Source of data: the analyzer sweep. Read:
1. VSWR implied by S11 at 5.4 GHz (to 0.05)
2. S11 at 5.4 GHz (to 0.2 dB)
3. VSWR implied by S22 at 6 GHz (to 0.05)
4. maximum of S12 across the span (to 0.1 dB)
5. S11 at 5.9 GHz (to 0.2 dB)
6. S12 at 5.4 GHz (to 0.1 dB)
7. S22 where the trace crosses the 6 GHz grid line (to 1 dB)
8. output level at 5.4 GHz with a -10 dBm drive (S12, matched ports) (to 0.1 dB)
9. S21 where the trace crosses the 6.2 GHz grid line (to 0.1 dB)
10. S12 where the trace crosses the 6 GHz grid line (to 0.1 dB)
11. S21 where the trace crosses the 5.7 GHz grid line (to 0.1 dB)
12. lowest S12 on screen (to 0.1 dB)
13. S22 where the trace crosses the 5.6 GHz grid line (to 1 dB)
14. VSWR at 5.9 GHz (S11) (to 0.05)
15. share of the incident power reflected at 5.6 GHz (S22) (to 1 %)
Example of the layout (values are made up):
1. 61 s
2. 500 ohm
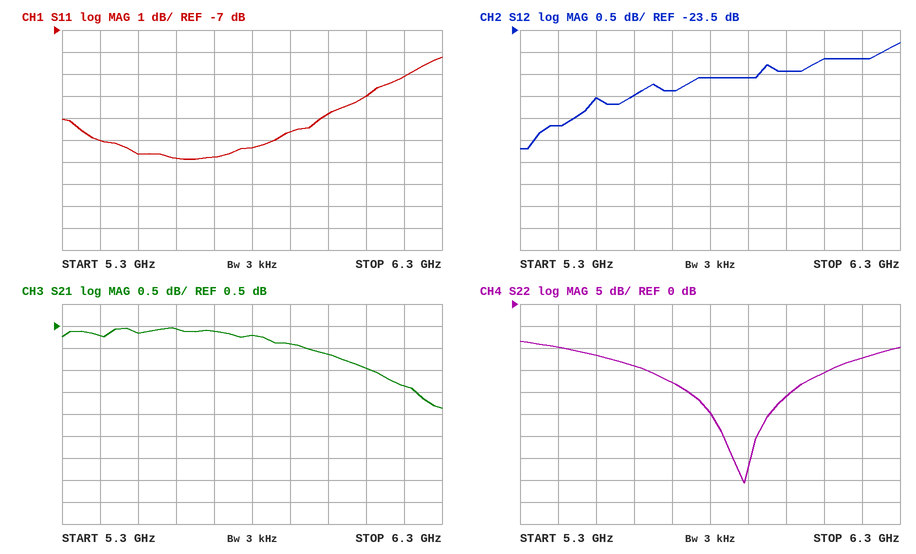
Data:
1. 1.65
2. -12.0 dB
3. 1.20
4. -23.8 dB
5. -11.6 dB
6. -25.7 dB
7. -21 dB
8. -35.7 dBm
9. -0.9 dB
10. -24.4 dB
11. 0.4 dB
12. -26.2 dB
13. -14 dB
14. 1.70
15. 4 %
